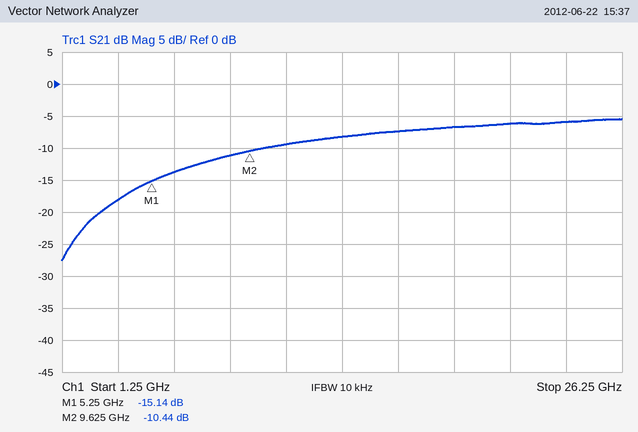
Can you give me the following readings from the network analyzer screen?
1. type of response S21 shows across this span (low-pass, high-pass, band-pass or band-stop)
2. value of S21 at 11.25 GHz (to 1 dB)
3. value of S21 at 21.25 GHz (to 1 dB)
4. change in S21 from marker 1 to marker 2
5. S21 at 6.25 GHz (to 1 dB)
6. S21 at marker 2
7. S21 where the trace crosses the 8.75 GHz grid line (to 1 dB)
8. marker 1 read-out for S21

high-pass
-9 dB
-6 dB
4.70 dB
-14 dB
-10.44 dB
-11 dB
-15.14 dB
